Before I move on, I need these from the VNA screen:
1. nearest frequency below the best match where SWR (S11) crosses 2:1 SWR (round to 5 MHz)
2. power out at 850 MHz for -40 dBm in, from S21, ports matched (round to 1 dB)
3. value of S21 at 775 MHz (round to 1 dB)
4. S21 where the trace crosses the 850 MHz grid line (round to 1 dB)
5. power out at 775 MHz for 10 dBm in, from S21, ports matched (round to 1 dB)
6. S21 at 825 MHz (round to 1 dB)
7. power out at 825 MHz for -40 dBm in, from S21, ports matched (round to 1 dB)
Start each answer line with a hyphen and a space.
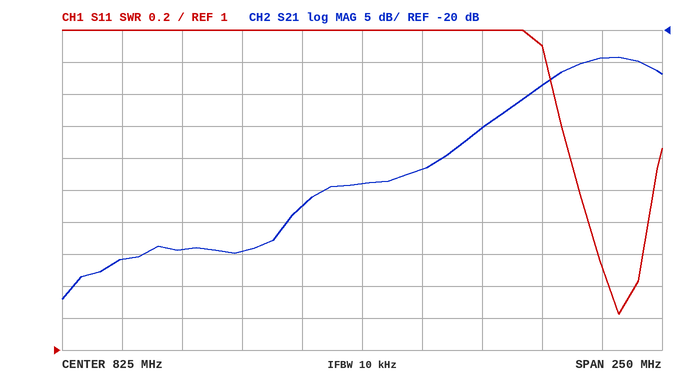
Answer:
- 915 MHz
- -82 dBm
- -55 dB
- -42 dB
- -45 dBm
- -44 dB
- -84 dBm
